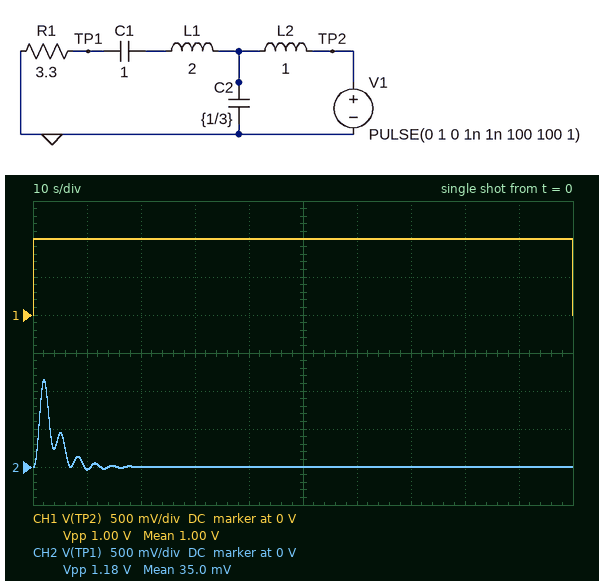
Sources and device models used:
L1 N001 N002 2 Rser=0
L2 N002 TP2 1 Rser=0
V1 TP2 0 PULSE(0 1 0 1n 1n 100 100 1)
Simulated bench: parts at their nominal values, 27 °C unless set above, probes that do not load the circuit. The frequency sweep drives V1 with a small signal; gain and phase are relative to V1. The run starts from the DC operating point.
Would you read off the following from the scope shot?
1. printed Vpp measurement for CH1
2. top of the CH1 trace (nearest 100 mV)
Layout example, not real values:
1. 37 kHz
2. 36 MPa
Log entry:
1. 1.00 V
2. 1.0 V
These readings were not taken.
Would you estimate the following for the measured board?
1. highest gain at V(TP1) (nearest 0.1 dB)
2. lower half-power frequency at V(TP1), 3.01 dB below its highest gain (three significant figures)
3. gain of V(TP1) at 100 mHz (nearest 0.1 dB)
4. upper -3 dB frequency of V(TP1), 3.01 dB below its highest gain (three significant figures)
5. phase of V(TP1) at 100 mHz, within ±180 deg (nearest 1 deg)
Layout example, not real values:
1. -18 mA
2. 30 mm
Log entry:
1. 7.7 dB
2. 262 mHz
3. 1.2 dB
4. 347 mHz
5. -7 deg
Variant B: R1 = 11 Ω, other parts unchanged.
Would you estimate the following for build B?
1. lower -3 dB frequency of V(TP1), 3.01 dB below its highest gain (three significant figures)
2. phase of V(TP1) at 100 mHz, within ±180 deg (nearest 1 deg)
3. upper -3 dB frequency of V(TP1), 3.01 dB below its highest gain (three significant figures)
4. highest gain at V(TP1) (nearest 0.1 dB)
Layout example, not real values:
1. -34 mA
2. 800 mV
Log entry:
1. 257 mHz
2. -2 deg
3. 300 mHz
4. 16.2 dB
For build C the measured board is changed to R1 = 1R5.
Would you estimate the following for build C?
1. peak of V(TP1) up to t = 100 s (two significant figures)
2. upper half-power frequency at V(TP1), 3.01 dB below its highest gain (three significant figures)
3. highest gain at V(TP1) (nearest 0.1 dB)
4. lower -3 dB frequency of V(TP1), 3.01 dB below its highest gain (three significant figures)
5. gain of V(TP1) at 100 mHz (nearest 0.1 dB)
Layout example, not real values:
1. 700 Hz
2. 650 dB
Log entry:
1. 740 mV
2. 356 mHz
3. 5.6 dB
4. 311 mHz
5. 0.9 dB
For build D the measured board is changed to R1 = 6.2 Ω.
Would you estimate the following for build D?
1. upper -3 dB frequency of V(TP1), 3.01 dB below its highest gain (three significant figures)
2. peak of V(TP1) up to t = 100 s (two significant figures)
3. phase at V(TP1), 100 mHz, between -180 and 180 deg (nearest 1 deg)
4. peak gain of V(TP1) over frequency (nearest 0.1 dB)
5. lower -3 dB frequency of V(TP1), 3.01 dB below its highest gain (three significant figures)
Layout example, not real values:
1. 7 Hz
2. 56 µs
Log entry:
1. 320 mHz
2. 1.4 V
3. -4 deg
4. 11.6 dB
5. 250 mHz
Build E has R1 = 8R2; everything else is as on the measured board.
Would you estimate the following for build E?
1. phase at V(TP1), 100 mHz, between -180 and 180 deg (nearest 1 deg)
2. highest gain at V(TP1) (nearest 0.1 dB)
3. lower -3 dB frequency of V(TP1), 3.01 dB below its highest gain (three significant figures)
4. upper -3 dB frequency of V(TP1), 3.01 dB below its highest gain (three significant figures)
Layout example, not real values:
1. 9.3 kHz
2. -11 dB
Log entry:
1. -3 deg
2. 13.8 dB
3. 253 mHz
4. 309 mHz
